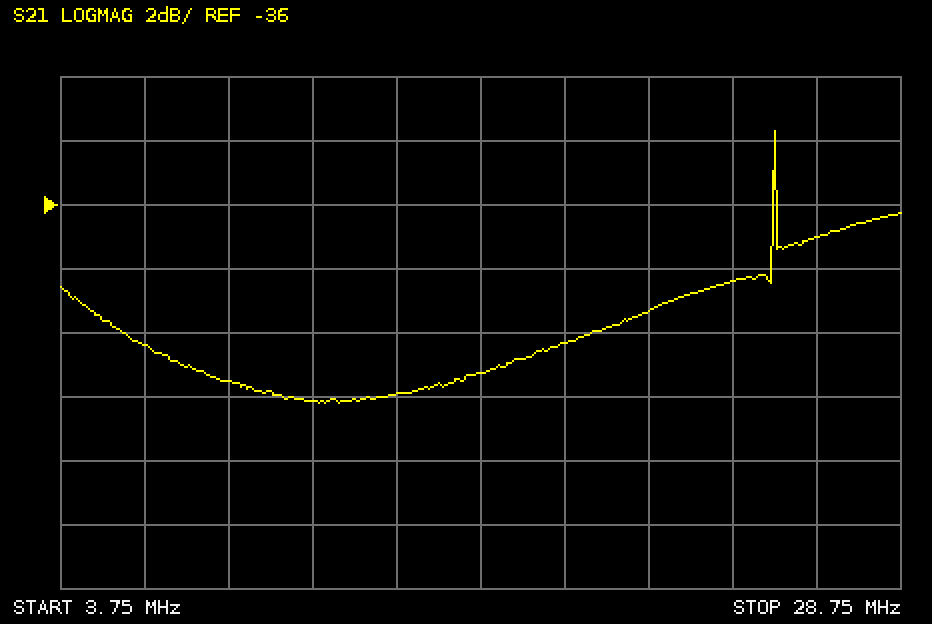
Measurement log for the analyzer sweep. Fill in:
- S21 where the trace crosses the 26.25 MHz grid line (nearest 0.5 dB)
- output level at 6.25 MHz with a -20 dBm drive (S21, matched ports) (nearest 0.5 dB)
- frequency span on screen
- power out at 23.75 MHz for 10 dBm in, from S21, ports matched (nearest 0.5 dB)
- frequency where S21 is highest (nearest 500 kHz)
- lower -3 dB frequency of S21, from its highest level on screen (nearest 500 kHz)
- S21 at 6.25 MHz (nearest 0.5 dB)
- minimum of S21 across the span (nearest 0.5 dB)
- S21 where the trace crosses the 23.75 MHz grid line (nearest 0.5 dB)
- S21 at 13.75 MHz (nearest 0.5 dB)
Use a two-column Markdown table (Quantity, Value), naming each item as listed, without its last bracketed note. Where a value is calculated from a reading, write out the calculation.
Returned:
| Quantity | Value |
|---|---|
| S21 where the trace crosses the 26.25 MHz grid line | -37.0 dB |
| output level at 6.25 MHz with a -20 dBm drive (S21, matched ports) | -20 dBm + (-40.5 dB) = -60.5 dBm |
| frequency span on screen | 25 MHz |
| power out at 23.75 MHz for 10 dBm in, from S21, ports matched | 10 dBm + (-38.5 dB) = -28.5 dBm |
| frequency where S21 is highest | 25.0 MHz |
| lower -3 dB frequency of S21, from its highest level on screen | 25.0 MHz |
| S21 at 6.25 MHz | -40.5 dB |
| minimum of S21 across the span | -42.0 dB |
| S21 where the trace crosses the 23.75 MHz grid line | -38.5 dB |
| S21 at 13.75 MHz | -42.0 dB |
